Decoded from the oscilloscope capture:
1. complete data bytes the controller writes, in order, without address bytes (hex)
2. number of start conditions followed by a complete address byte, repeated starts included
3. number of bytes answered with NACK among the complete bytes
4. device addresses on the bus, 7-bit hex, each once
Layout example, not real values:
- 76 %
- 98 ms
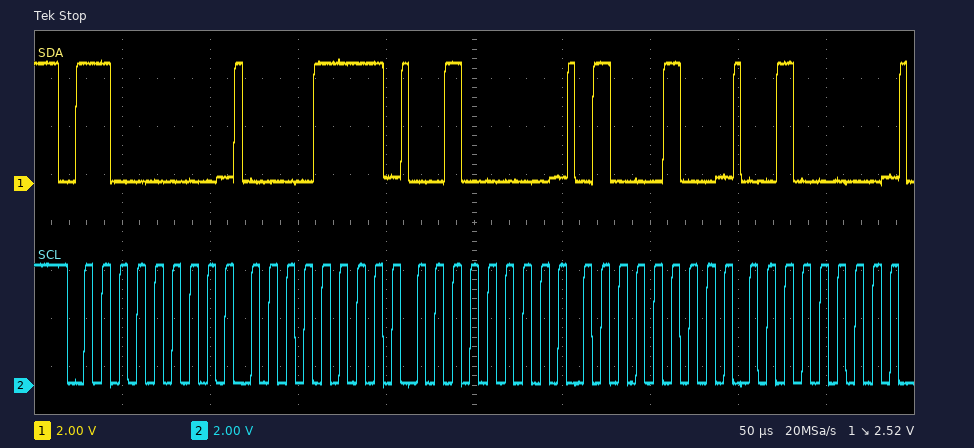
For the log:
- 0F 20 44 20
- 1
- 0
- 0x60
